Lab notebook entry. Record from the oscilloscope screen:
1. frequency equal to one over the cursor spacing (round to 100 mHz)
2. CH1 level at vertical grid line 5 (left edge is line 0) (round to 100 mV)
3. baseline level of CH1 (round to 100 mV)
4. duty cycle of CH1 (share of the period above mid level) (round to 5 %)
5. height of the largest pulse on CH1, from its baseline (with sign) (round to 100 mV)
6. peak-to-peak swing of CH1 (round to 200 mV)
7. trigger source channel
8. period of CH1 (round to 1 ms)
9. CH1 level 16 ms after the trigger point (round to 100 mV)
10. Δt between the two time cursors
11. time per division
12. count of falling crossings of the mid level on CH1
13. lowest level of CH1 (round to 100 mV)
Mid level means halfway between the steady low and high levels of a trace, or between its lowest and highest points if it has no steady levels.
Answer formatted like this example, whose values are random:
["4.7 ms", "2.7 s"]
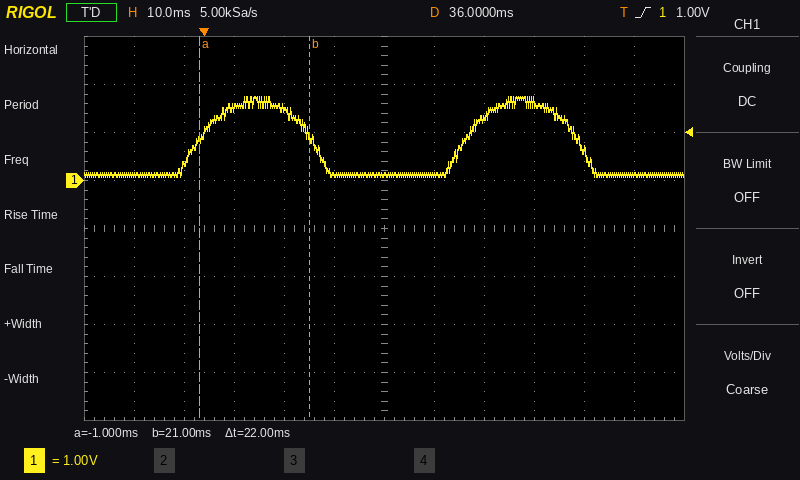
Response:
["45.5 Hz", "100 mV", "100 mV", "40 %", "+1.6 V", "1.6 V", "CH1", "53 ms", "1.5 V", "22 ms", "10 ms", "2", "100 mV"]
